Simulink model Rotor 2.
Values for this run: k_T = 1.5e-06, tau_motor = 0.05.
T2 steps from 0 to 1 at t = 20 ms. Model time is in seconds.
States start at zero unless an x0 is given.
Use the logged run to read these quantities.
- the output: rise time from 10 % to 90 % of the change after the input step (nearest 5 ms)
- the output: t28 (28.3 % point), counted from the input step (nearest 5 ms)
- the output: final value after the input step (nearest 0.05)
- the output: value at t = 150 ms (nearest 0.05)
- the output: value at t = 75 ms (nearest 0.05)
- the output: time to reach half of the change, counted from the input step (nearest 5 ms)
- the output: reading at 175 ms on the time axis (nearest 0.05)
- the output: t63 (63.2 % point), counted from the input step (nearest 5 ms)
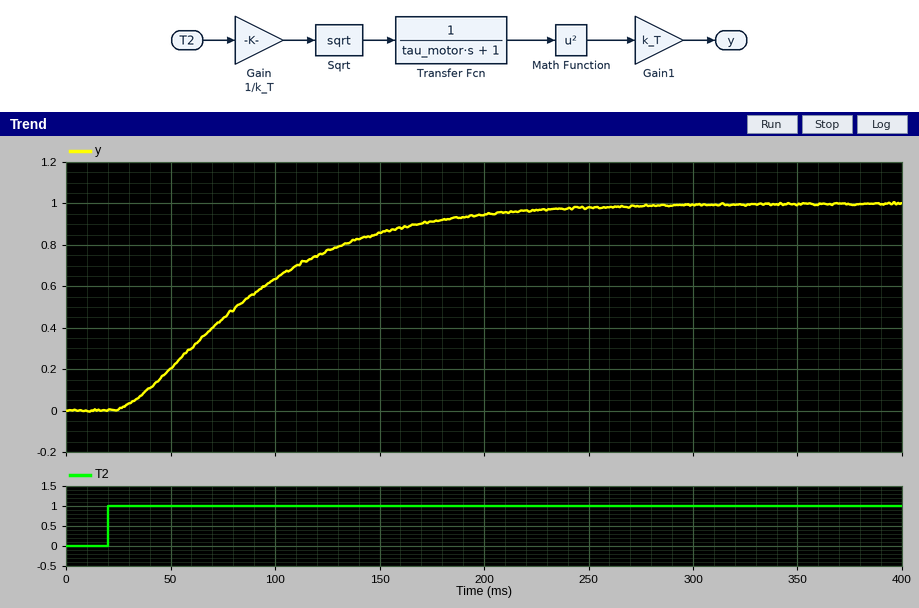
130 ms
40 ms
1.00
0.85
0.45
60 ms
0.90
80 ms
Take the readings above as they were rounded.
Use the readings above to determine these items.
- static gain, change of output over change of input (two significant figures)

1.0
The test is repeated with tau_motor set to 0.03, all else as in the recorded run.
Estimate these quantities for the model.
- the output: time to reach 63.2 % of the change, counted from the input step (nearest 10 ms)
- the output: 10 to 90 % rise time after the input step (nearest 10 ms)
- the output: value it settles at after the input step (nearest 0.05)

50 ms
80 ms
1.00
